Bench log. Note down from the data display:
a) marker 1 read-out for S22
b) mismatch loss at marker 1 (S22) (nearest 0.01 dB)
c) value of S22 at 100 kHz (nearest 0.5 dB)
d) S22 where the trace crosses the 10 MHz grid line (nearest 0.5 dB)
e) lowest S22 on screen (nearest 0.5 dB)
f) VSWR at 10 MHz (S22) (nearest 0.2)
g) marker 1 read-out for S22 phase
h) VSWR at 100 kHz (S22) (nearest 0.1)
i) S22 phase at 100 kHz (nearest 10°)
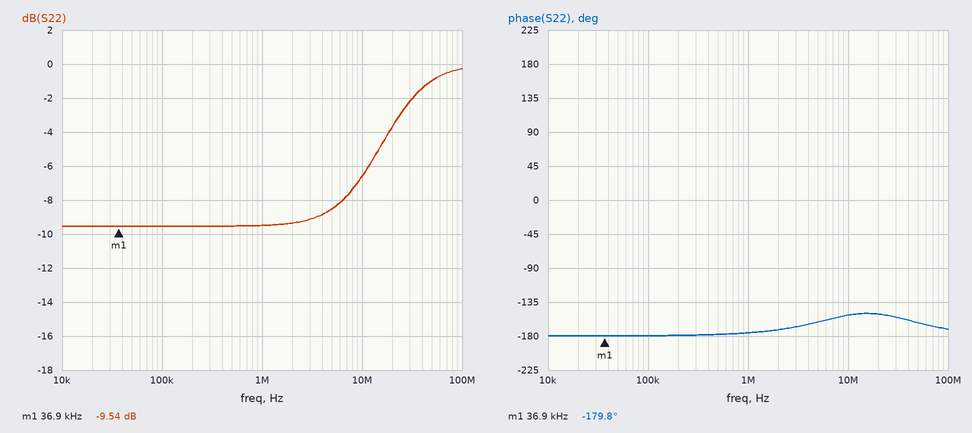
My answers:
-9.54 dB
0.51 dB
-9.5 dB
-6.5 dB
-9.5 dB
2.8
-179.8°
2.0
-180°
